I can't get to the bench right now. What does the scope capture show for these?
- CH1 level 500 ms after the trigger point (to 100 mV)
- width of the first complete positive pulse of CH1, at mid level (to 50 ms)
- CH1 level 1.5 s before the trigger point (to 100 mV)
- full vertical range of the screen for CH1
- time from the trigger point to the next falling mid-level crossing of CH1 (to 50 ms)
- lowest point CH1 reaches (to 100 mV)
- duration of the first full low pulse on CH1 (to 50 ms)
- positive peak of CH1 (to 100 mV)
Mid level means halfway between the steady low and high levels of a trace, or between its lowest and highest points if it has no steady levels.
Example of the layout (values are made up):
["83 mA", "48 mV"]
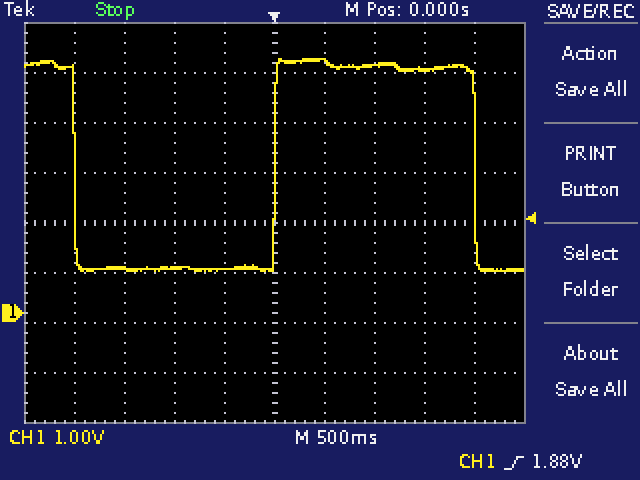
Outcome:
["5.0 V", "2.00 s", "900 mV", "8 V", "2.00 s", "800 mV", "2.00 s", "5.1 V"]
